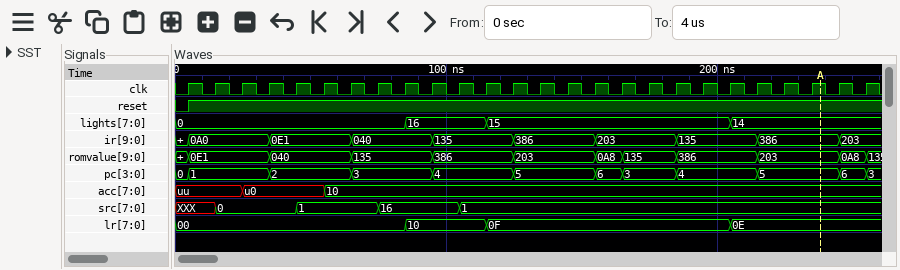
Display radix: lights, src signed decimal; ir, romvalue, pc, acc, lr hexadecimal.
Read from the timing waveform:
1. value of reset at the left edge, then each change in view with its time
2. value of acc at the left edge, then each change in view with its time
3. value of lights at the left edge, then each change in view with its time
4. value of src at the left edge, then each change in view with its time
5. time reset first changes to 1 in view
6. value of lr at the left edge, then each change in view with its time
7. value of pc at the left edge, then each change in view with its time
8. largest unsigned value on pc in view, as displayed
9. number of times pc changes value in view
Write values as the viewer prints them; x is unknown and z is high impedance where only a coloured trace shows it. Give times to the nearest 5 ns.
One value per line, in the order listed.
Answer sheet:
0, 1 at 5 ns
uu, u0 at 25 ns, 10 at 55 ns
0, 16 at 85 ns, 15 at 115 ns, 14 at 205 ns
XXX, 0 at 15 ns, 1 at 45 ns, 16 at 75 ns, 1 at 105 ns
5 ns
00, 10 at 85 ns, 0F at 115 ns, 0E at 205 ns
0, 1 at 5 ns, 2 at 35 ns, 3 at 65 ns, 4 at 95 ns, 5 at 125 ns, 6 at 155 ns, 3 at 165 ns, 4 at 185 ns, 5 at 215 ns, 6 at 245 ns, 3 at 255 ns
6
11
